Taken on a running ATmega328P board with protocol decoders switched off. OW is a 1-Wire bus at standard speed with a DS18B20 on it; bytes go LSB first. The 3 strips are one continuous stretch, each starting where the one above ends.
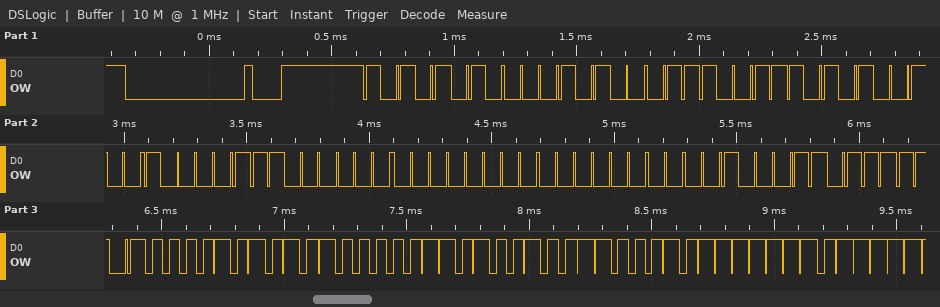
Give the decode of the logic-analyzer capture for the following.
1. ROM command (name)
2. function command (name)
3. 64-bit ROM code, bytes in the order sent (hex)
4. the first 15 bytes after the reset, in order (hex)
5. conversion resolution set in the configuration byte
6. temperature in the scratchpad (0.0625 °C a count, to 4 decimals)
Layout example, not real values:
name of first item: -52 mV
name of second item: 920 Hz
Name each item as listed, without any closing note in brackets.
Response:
ROM command: Match ROM
function command: Read Scratchpad
64-bit ROM code, bytes in the order sent: 28 CE 95 84 03 00 00 C4
the first 15 bytes after the reset, in order: 55 28 CE 95 84 03 00 00 C4 BE 50 05 4B 46 7F
conversion resolution set in the configuration byte: 12 bits
temperature in the scratchpad: 85.0000 °C
